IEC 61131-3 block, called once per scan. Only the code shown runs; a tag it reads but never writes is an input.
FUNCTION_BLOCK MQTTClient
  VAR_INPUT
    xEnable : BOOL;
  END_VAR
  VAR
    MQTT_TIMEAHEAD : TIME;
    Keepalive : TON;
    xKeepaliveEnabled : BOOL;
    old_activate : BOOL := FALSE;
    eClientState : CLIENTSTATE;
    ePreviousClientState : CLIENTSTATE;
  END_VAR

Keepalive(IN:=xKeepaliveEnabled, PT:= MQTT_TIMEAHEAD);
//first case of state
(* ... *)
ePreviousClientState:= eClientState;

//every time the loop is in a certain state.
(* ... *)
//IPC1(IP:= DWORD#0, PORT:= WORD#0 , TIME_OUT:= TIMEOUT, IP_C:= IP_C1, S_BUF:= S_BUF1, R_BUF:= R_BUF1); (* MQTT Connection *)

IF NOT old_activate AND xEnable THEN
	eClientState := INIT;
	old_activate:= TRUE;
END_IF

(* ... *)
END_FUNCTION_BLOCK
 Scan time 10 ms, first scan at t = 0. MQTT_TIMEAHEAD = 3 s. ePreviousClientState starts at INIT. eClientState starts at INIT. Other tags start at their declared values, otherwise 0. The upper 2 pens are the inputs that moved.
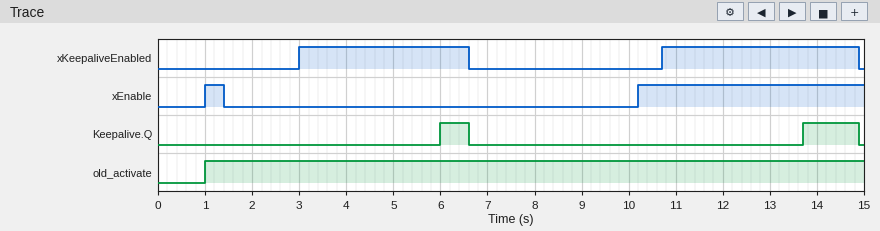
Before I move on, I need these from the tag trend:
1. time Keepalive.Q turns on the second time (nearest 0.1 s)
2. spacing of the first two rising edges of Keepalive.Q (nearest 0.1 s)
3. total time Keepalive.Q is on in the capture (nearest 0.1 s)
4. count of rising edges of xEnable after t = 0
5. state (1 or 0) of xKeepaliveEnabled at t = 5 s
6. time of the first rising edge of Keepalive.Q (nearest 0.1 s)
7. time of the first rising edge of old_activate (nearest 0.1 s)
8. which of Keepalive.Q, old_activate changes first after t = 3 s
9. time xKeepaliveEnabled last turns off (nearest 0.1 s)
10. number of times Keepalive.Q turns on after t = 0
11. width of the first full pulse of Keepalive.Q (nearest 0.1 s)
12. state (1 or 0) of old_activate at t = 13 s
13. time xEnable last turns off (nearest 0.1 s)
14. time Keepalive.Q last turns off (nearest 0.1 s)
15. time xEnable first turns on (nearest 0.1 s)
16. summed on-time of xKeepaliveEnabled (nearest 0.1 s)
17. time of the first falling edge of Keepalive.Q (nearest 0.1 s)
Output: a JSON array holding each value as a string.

["13.7 s", "7.7 s", "1.8 s", "2", "1", "6.0 s", "1.0 s", "Keepalive.Q", "14.9 s", "2", "0.6 s", "1", "1.4 s", "14.9 s", "1.0 s", "7.8 s", "6.6 s"]
